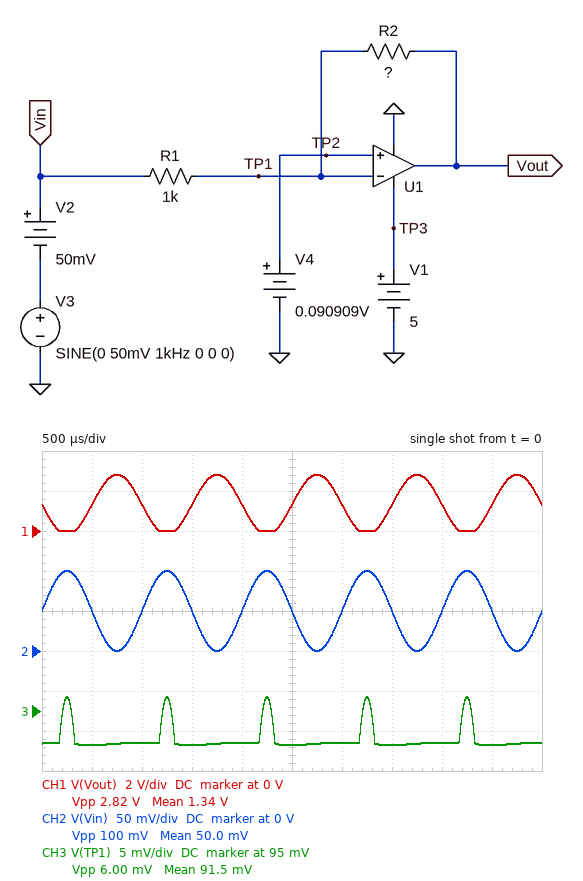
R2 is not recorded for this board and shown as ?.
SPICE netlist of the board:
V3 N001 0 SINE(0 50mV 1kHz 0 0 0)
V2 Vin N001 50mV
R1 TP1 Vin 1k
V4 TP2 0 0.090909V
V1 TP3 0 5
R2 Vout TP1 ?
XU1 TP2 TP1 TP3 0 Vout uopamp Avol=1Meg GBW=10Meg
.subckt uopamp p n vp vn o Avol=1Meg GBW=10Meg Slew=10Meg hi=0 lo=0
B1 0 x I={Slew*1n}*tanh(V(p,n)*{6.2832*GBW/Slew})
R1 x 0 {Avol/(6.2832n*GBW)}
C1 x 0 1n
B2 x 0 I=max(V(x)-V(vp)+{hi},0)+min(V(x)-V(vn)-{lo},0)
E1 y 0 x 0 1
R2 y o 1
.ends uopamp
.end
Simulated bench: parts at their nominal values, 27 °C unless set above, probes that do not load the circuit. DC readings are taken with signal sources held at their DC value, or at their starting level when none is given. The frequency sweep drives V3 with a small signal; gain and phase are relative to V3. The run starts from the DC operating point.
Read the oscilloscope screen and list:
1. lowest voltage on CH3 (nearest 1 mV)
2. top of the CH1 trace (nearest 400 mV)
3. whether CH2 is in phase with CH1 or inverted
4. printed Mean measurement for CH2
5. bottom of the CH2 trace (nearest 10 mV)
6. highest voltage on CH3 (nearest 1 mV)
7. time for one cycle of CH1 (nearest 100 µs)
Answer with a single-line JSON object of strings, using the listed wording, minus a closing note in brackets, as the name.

{"lowest voltage on CH3": "91 mV", "top of the CH1 trace": "2.8 V", "whether CH2 is in phase with CH1 or inverted": "inverted", "printed Mean measurement for CH2": "50.0 mV", "bottom of the CH2 trace": "0 V", "highest voltage on CH3": "97 mV", "time for one cycle of CH1": "1.0 ms"}
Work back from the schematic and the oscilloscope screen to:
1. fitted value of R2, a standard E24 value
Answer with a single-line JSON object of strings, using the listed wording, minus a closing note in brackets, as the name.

{"fitted value of R2, a standard E24 value": "30 kΩ"}
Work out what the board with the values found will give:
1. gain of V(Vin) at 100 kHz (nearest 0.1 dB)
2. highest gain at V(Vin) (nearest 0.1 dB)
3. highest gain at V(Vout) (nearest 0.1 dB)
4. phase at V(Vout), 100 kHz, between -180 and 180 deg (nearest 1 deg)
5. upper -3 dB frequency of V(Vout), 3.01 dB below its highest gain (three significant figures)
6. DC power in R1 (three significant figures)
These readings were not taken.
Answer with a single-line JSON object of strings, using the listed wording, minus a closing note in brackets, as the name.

{"gain of V(Vin) at 100 kHz": "0 dB", "highest gain at V(Vin)": "0 dB", "highest gain at V(Vout)": "29.5 dB", "phase at V(Vout), 100 kHz, between -180 and 180 deg": "163 deg", "upper -3 dB frequency of V(Vout), 3.01 dB below its highest gain": "323 kHz", "DC power in R1": "1.67 µW"}
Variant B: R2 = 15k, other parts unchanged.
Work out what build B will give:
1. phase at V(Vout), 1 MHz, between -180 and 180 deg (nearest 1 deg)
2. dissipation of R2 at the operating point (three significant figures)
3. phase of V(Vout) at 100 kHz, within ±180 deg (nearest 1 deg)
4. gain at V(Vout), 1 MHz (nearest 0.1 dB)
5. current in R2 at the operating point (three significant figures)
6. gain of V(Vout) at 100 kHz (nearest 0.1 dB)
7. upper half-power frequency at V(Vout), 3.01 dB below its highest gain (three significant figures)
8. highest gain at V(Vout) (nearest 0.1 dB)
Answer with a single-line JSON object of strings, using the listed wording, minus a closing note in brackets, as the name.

{"phase at V(Vout), 1 MHz, between -180 and 180 deg": "122 deg", "dissipation of R2 at the operating point": "25.1 µW", "phase of V(Vout) at 100 kHz, within ±180 deg": "171 deg", "gain at V(Vout), 1 MHz": "18.0 dB", "current in R2 at the operating point": "40.9 µA", "gain of V(Vout) at 100 kHz": "23.4 dB", "upper half-power frequency at V(Vout), 3.01 dB below its highest gain": "625 kHz", "highest gain at V(Vout)": "23.5 dB"}
